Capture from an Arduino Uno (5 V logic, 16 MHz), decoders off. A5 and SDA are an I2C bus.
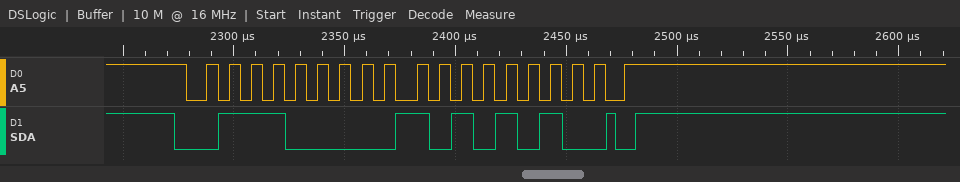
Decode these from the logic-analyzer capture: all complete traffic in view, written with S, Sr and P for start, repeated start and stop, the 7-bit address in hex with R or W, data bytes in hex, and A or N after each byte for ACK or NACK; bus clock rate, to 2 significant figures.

S 38W A AA A P
100 kHz
